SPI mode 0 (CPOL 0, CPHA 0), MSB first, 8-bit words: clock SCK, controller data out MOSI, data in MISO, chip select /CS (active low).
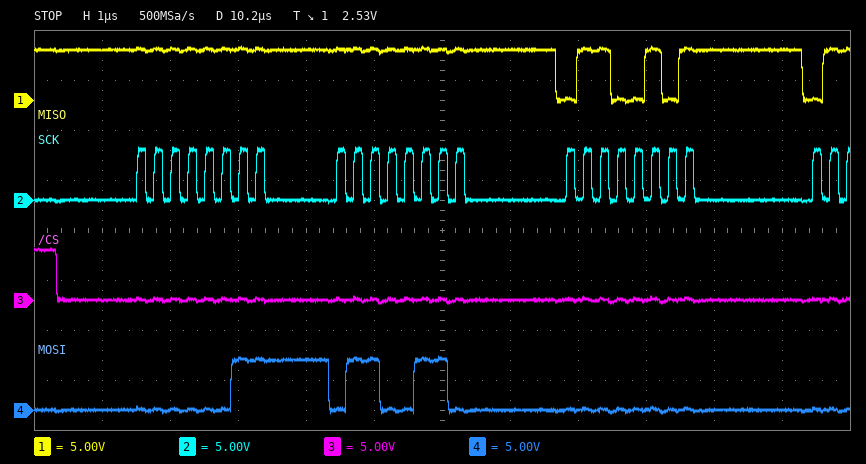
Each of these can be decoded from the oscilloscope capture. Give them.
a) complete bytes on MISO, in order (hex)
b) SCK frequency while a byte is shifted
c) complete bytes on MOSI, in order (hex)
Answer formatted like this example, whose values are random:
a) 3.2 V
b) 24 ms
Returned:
a) 0xFF 0xFF 0x65
b) 4 MHz
c) 0x03 0x66 0x00
